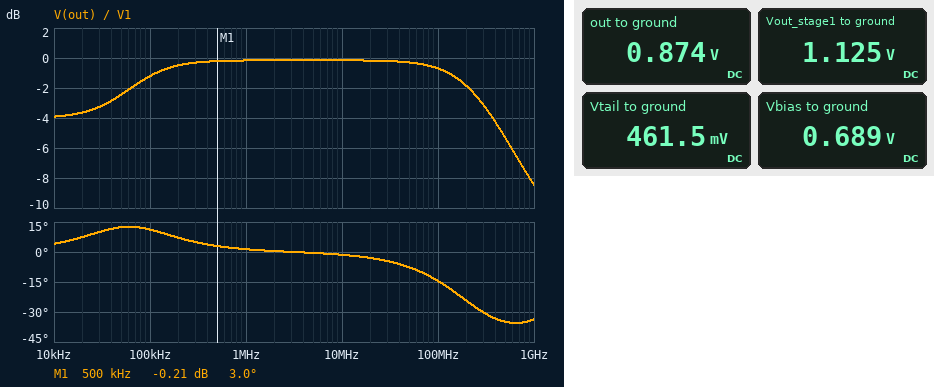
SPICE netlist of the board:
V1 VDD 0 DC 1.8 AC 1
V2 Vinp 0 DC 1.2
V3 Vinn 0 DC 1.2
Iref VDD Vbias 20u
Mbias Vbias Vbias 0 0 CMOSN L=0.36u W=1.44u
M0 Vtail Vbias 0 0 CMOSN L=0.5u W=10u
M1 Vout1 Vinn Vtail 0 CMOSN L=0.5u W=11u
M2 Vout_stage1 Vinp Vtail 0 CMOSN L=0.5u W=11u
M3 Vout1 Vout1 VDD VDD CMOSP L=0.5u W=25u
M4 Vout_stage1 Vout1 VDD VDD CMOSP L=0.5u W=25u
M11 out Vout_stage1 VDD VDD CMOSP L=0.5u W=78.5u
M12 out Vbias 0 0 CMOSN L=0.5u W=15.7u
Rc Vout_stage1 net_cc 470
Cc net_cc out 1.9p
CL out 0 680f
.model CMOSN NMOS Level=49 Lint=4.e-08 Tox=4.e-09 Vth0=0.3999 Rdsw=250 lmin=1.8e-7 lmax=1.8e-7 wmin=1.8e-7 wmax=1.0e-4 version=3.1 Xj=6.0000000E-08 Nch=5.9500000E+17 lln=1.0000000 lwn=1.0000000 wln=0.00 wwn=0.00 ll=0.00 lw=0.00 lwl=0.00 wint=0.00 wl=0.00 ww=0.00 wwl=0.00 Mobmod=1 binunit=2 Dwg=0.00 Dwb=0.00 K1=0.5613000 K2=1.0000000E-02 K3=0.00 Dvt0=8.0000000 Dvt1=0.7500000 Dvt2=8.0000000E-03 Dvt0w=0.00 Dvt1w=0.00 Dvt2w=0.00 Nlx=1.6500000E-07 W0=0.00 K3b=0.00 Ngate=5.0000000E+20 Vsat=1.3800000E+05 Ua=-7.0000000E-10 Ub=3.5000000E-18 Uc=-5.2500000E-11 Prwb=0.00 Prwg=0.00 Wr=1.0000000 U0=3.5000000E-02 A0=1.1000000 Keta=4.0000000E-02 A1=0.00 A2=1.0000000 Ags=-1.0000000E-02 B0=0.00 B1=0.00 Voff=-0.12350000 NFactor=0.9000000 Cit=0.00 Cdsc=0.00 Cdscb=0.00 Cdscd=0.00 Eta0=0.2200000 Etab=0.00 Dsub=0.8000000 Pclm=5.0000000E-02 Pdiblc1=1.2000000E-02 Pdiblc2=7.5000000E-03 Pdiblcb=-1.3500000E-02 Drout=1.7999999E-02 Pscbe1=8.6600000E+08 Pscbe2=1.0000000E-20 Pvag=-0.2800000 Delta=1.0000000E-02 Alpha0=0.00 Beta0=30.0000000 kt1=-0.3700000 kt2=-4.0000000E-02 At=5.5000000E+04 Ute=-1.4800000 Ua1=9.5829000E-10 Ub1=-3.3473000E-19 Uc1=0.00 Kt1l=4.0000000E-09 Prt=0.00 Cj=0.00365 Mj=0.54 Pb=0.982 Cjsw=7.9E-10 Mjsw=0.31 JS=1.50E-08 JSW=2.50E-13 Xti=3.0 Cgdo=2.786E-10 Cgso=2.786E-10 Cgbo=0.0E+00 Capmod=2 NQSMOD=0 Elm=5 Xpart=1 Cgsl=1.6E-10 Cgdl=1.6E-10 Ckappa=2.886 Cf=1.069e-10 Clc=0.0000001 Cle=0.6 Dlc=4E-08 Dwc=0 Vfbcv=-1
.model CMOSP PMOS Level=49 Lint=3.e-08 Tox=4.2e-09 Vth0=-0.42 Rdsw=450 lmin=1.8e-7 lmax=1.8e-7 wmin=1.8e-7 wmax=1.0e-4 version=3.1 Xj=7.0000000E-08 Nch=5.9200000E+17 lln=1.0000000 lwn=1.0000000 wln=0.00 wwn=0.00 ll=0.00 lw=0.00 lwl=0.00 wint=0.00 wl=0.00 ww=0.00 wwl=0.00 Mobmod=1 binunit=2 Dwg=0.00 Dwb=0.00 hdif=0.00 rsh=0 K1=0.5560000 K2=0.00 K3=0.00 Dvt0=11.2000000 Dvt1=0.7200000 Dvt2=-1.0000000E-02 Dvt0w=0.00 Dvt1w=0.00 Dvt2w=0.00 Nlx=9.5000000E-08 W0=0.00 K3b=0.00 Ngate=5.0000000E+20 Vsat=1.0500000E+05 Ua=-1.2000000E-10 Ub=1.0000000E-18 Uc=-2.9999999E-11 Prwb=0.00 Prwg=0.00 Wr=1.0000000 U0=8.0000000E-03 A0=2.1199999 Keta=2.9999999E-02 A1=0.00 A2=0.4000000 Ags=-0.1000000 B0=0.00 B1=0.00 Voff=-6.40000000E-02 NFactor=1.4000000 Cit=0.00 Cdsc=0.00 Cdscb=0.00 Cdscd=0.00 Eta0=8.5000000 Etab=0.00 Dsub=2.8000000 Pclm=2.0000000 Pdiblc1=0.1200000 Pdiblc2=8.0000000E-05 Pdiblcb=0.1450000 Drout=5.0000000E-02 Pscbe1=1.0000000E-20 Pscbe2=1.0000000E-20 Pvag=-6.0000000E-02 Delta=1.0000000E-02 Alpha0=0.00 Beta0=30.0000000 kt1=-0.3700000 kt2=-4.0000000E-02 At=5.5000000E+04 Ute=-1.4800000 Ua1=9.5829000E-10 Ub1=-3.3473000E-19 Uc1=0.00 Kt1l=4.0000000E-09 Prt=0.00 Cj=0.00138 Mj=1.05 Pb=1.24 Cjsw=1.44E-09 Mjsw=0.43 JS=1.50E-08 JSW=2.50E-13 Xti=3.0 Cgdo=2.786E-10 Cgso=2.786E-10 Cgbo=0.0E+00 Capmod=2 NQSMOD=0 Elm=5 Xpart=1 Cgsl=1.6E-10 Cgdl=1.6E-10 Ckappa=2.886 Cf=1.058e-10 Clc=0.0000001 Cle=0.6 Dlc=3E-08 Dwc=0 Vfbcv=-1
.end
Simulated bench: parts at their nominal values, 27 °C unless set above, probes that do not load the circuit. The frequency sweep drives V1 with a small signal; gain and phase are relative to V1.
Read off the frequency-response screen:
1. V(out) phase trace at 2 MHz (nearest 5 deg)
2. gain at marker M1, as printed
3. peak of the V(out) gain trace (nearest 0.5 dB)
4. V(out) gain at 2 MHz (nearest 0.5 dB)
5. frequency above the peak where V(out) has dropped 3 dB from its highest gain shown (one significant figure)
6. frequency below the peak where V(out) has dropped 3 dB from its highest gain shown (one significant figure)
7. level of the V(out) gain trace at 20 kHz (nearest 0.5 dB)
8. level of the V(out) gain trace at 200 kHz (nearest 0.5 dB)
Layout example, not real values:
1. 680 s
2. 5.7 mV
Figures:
1. 0 deg
2. -0.21 dB
3. 0 dB
4. 0 dB
5. 300 MHz
6. 30 kHz
7. -3.5 dB
8. -0.5 dB
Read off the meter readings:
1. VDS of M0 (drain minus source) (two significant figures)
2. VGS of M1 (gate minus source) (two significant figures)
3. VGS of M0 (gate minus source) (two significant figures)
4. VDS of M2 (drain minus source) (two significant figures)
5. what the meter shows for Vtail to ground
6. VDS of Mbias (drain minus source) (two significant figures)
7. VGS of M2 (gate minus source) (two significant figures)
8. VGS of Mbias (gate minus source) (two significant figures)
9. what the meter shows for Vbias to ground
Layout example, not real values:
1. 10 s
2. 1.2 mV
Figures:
1. 460 mV
2. 740 mV
3. 690 mV
4. 660 mV
5. 461.5 mV
6. 690 mV
7. 740 mV
8. 690 mV
9. 0.689 V
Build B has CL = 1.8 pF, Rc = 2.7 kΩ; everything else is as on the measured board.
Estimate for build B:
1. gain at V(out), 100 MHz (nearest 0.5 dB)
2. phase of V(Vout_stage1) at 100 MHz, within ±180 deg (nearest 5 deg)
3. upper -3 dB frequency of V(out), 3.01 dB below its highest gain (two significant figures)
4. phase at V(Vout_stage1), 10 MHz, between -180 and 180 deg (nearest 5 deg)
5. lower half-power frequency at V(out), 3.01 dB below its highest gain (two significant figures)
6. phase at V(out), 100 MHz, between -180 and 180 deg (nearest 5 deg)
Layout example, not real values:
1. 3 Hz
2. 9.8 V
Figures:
1. -1.5 dB
2. -25 deg
3. 140 MHz
4. -5 deg
5. 31 kHz
6. -45 deg
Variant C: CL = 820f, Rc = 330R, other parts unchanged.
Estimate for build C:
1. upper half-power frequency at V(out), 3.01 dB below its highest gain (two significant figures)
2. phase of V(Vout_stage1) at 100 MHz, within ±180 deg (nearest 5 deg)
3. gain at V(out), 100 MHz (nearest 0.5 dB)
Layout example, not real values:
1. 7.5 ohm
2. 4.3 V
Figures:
1. 250 MHz
2. -15 deg
3. -1.0 dB
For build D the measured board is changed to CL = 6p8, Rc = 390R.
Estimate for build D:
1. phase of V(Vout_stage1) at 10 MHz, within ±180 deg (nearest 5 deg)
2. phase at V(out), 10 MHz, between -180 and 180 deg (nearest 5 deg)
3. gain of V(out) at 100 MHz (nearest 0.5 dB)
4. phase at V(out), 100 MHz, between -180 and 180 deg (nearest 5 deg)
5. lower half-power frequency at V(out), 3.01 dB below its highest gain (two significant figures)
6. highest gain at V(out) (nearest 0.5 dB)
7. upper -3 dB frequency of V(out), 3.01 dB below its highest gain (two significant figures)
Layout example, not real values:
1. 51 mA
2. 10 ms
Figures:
1. -10 deg
2. -15 deg
3. -9.0 dB
4. -60 deg
5. 25 kHz
6. -0.5 dB
7. 40 MHz
